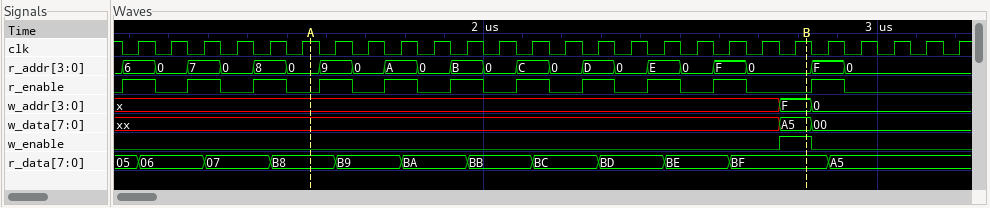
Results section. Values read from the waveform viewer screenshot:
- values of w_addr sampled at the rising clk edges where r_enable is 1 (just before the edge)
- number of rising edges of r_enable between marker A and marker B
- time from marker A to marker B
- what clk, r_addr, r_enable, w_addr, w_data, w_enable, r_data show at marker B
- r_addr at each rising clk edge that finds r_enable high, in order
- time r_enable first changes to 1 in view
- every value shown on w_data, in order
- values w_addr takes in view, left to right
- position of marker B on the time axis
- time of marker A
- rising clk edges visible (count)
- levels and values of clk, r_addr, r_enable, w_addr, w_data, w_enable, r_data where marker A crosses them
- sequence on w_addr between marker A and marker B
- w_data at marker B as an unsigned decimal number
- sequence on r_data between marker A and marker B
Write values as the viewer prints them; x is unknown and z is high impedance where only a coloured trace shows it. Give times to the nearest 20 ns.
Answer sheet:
x, x, x, x, x, x, x, x, x, x, 0
7
1260 ns
clk=1, r_addr=0, r_enable=0, w_addr=F, w_data=A5, w_enable=1, r_data=BF
6, 7, 8, 9, A, B, C, D, E, F, F
1080 ns
xx, A5, 00
x, F, 0
2820 ns
1560 ns
26
clk=1, r_addr=0, r_enable=0, w_addr=x, w_data=xx, w_enable=0, r_data=B8
x, F
165
B8, B9, BA, BB, BC, BD, BE, BF
